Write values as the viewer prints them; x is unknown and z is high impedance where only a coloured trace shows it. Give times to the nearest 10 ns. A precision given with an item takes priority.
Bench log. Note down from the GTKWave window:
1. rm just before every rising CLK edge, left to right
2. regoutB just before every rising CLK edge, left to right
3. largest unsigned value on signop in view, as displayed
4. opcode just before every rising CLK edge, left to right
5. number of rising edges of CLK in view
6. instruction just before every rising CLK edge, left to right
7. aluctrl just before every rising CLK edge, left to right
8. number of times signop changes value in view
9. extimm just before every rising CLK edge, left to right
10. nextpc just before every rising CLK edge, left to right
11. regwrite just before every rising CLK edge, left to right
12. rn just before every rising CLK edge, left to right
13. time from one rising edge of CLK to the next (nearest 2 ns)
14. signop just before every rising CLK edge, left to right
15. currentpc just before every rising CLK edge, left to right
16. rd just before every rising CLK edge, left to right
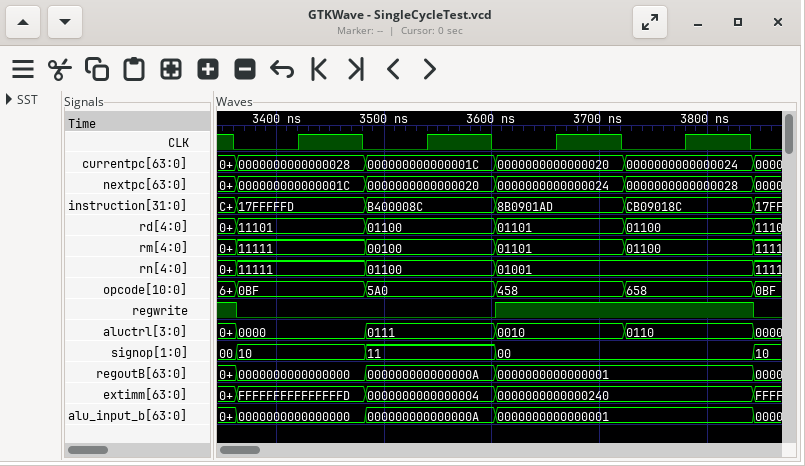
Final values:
11111, 00100, 01101, 01100
0000000000000000, 000000000000000A, 0000000000000001, 0000000000000001
11
0BF, 5A0, 458, 658
4
17FFFFFD, B400008C, 8B0901AD, CB09018C
0000, 0111, 0010, 0110
4
FFFFFFFFFFFFFFFD, 0000000000000004, 0000000000000240, 0000000000000240
000000000000001C, 0000000000000020, 0000000000000024, 0000000000000028
0 0 1 1
11111, 01100, 01001, 01001
120 ns
10, 11, 00, 00
0000000000000028, 000000000000001C, 0000000000000020, 0000000000000024
11101, 01100, 01101, 01100
